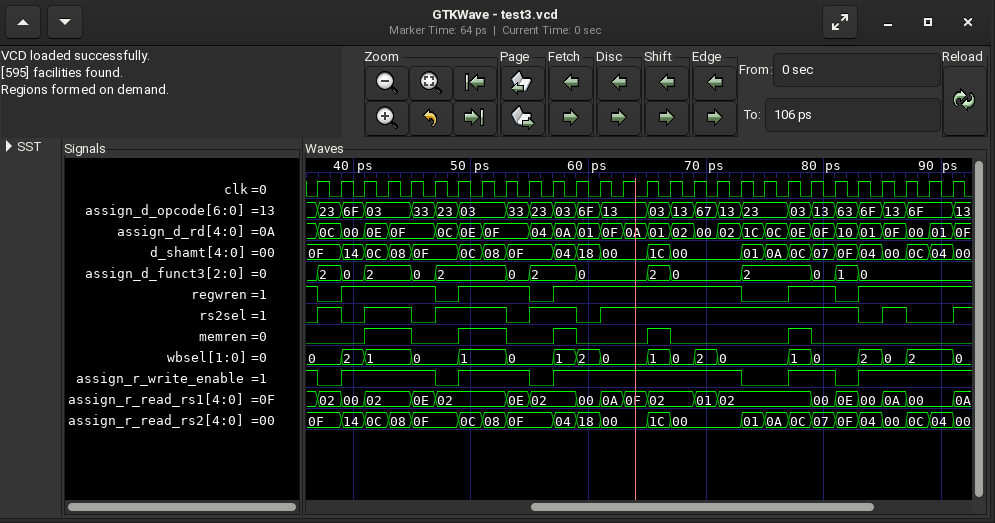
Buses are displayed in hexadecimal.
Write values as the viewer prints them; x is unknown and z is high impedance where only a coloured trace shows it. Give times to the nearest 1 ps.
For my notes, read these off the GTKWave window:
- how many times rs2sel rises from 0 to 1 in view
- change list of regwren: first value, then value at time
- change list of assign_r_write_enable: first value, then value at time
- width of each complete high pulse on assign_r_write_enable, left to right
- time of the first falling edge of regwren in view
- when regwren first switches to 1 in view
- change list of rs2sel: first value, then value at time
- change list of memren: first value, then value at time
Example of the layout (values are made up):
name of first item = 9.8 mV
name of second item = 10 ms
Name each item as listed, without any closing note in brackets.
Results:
how many times rs2sel rises from 0 to 1 in view = 7
change list of regwren: first value, then value at time = 1, 0 at 37 ps, 1 at 39 ps, 0 at 47 ps, 1 at 49 ps, 0 at 55 ps, 1 at 57 ps, 0 at 73 ps, 1 at 77 ps, 0 at 81 ps, 1 at 83 ps
change list of assign_r_write_enable: first value, then value at time = 1, 0 at 37 ps, 1 at 39 ps, 0 at 47 ps, 1 at 49 ps, 0 at 55 ps, 1 at 57 ps, 0 at 73 ps, 1 at 77 ps, 0 at 81 ps, 1 at 83 ps
width of each complete high pulse on assign_r_write_enable, left to right = 8 ps, 6 ps, 16 ps, 4 ps
time of the first falling edge of regwren in view = 37 ps
when regwren first switches to 1 in view = 39 ps
change list of rs2sel: first value, then value at time = 0, 1 at 37 ps, 0 at 39 ps, 1 at 41 ps, 0 at 45 ps, 1 at 47 ps, 0 at 53 ps, 1 at 55 ps, 0 at 59 ps, 1 at 61 ps, 0 at 83 ps, 1 at 85 ps, 0 at 87 ps, 1 at 91 ps
change list of memren: first value, then value at time = 0, 1 at 41 ps, 0 at 45 ps, 1 at 49 ps, 0 at 53 ps, 1 at 57 ps, 0 at 59 ps, 1 at 65 ps, 0 at 67 ps, 1 at 77 ps, 0 at 79 ps
